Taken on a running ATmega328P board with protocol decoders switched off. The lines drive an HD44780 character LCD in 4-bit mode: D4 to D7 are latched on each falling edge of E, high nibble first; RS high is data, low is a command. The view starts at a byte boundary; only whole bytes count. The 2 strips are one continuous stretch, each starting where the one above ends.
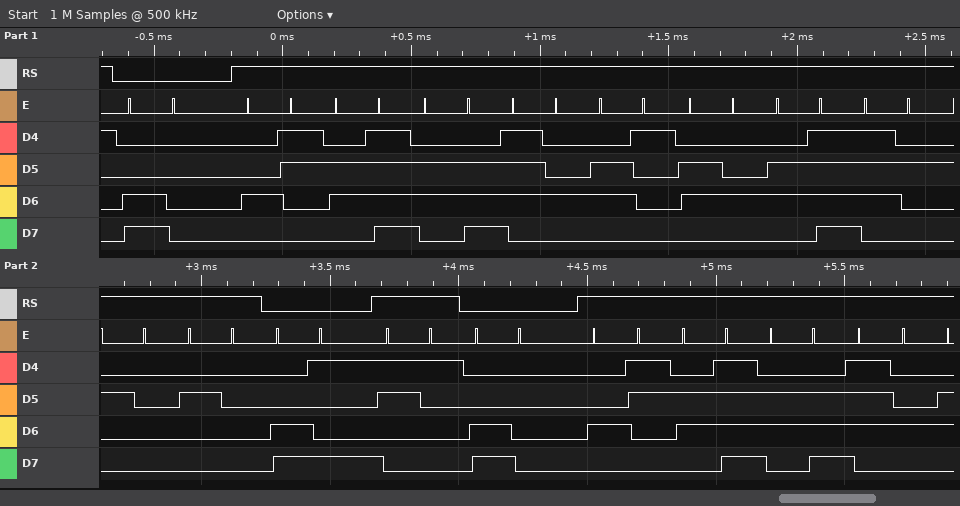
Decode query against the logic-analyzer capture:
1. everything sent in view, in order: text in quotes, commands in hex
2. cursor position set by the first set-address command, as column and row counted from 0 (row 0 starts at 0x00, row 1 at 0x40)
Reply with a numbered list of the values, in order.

1. 0xC0 "Contador  " 0xC9 "1" 0xC0 "Cont"
2. column 0, row 1
